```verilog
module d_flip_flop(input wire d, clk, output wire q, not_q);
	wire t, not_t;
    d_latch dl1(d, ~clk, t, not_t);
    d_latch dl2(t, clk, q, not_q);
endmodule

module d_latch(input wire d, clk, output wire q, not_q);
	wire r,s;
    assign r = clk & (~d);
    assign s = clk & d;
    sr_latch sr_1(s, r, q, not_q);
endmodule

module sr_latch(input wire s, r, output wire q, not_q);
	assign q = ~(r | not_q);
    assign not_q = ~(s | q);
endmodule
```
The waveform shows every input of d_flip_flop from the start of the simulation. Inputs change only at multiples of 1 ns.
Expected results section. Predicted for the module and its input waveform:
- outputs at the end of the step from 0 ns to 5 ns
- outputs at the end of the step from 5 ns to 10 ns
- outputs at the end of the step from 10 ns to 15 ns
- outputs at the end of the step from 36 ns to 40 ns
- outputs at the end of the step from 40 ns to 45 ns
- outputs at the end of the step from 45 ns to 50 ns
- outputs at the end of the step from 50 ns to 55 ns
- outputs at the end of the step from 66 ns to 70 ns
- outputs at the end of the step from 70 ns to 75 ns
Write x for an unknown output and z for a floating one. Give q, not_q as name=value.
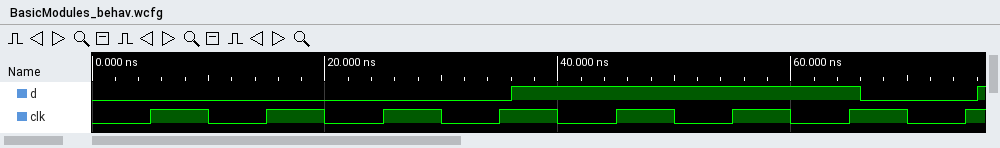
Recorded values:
q=x, not_q=x
q=0, not_q=1
q=0, not_q=1
q=0, not_q=1
q=0, not_q=1
q=1, not_q=0
q=1, not_q=0
q=1, not_q=0
q=1, not_q=0
